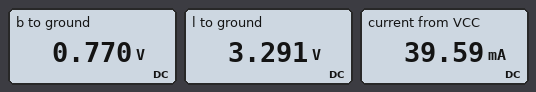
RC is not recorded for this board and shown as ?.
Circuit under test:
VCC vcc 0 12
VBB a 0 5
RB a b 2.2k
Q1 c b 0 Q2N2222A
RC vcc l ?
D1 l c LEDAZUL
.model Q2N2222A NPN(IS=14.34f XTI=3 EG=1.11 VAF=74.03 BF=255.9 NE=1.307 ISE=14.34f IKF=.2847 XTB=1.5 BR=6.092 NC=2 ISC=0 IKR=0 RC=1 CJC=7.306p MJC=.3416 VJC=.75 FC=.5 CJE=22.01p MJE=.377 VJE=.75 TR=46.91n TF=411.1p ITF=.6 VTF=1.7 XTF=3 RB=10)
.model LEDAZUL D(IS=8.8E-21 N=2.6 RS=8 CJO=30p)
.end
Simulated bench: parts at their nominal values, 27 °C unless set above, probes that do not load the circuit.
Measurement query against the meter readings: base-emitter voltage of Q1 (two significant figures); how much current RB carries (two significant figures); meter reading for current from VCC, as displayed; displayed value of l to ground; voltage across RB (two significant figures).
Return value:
770 mV
1.9 mA
39.59 mA
3.291 V
4.2 V
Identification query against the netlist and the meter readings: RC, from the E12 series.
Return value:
220 Ω
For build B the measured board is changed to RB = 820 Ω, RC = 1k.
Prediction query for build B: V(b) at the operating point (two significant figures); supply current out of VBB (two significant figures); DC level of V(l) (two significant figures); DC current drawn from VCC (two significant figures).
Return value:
800 mV
5.1 mA
2.9 V
9.1 mA
